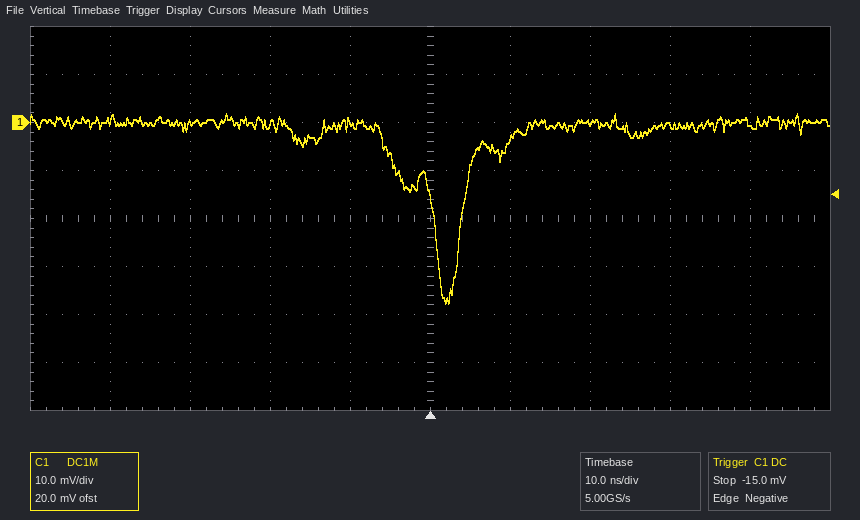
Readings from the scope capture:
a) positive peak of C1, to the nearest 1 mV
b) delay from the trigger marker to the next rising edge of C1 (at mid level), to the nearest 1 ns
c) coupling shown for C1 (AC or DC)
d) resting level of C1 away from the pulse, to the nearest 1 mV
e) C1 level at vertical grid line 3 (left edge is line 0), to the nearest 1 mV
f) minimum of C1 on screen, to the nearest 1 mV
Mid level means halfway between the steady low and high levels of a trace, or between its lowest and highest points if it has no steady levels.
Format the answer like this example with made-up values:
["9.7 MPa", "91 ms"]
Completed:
["2 mV", "4 ns", "DC", "0 mV", "0 mV", "-38 mV"]
